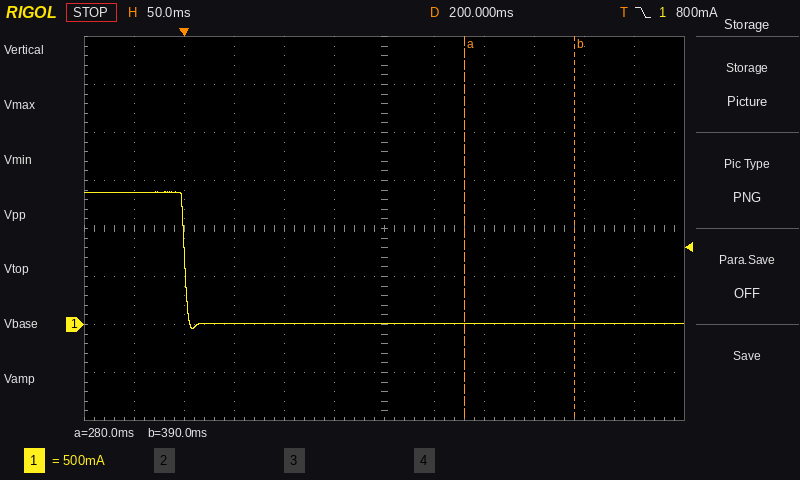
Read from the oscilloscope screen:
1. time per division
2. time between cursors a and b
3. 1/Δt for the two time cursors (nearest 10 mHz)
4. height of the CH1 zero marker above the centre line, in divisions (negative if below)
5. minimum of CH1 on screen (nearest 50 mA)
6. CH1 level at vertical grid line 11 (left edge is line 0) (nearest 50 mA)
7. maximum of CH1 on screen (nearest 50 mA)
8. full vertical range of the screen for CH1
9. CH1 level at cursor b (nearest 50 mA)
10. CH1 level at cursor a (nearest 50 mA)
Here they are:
50 ms
110 ms
9.09 Hz
-2.0 div
-50 mA
0 mA
1.40 A
4 A
0 mA
0 mA
